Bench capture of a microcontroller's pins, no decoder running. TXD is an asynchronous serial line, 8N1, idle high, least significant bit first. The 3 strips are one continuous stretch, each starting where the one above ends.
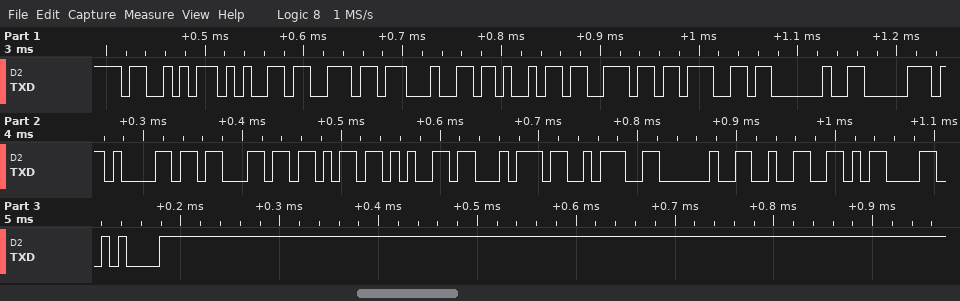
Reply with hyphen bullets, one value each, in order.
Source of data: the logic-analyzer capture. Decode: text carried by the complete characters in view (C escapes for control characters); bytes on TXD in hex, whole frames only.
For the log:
- "Sending packet: 2\r\n"
- 0x53 0x65 0x6E 0x64 0x69 0x6E 0x67 0x20 0x70 0x61 0x63 0x6B 0x65 0x74 0x3A 0x20 0x32 0x0D 0x0A
